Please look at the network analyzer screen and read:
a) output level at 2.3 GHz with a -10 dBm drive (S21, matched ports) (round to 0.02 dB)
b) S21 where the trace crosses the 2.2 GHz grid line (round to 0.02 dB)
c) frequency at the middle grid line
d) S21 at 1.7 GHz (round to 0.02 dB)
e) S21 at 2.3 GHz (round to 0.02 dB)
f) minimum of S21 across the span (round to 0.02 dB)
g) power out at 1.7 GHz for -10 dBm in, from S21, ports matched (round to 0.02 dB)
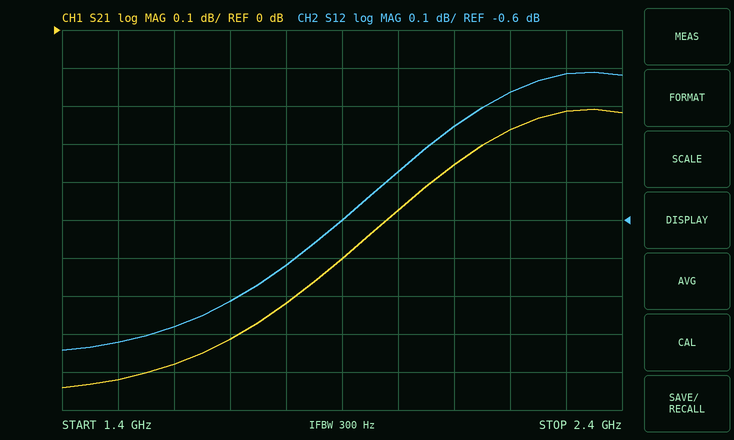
-10.22 dBm
-0.26 dB
1.9 GHz
-0.82 dB
-0.22 dB
-0.94 dB
-10.82 dBm
